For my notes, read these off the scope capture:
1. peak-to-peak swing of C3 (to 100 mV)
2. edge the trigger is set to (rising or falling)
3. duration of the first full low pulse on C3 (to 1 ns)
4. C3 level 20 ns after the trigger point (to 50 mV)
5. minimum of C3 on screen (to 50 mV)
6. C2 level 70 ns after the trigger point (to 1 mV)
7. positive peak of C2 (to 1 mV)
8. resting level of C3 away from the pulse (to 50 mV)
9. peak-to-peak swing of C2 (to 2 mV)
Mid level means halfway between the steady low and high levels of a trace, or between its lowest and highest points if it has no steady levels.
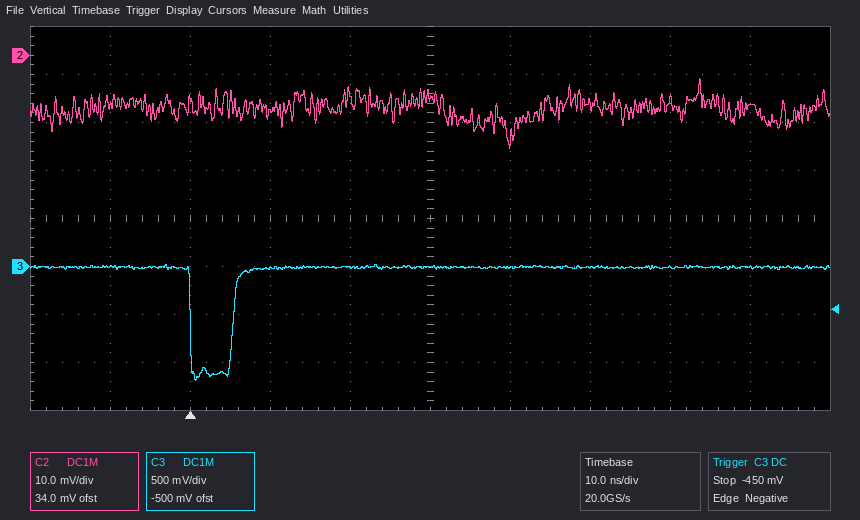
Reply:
1.20 V
falling
5 ns
0 mV
-1.20 V
-11 mV
-5 mV
0 mV
14 mV
